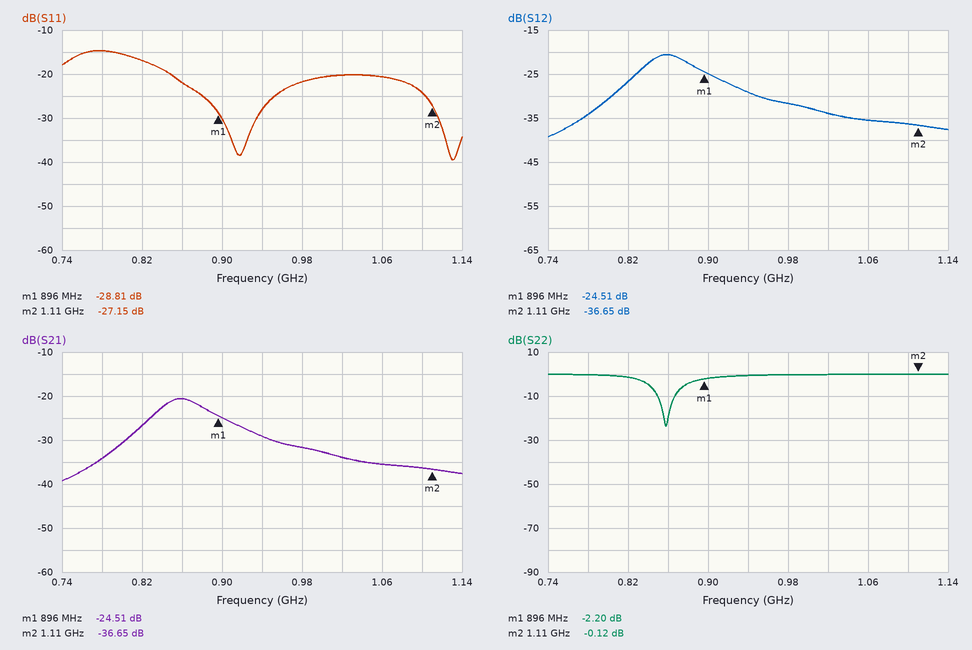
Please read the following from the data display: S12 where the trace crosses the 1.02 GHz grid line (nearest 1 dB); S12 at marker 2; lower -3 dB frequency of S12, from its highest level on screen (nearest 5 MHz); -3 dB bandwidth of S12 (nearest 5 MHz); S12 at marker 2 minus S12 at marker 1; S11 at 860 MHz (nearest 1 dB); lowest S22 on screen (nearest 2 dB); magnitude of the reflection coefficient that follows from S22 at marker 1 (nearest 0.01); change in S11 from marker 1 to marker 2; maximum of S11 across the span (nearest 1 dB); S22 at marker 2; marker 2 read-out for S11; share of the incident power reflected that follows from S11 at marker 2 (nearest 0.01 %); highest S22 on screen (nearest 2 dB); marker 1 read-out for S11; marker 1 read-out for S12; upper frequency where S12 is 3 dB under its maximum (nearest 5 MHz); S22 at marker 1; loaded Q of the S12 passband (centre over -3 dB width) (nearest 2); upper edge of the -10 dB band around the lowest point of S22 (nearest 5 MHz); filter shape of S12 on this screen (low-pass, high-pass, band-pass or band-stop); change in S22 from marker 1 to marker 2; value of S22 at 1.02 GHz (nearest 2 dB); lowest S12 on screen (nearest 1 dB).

-34 dB
-36.65 dB
835 MHz
55 MHz
-12.14 dB
-22 dB
-24 dB
0.78
1.66 dB
-15 dB
-0.12 dB
-27.15 dB
0.19 %
0 dB
-28.81 dB
-24.51 dB
890 MHz
-2.20 dB
16
865 MHz
band-pass
2.08 dB
0 dB
-39 dB
